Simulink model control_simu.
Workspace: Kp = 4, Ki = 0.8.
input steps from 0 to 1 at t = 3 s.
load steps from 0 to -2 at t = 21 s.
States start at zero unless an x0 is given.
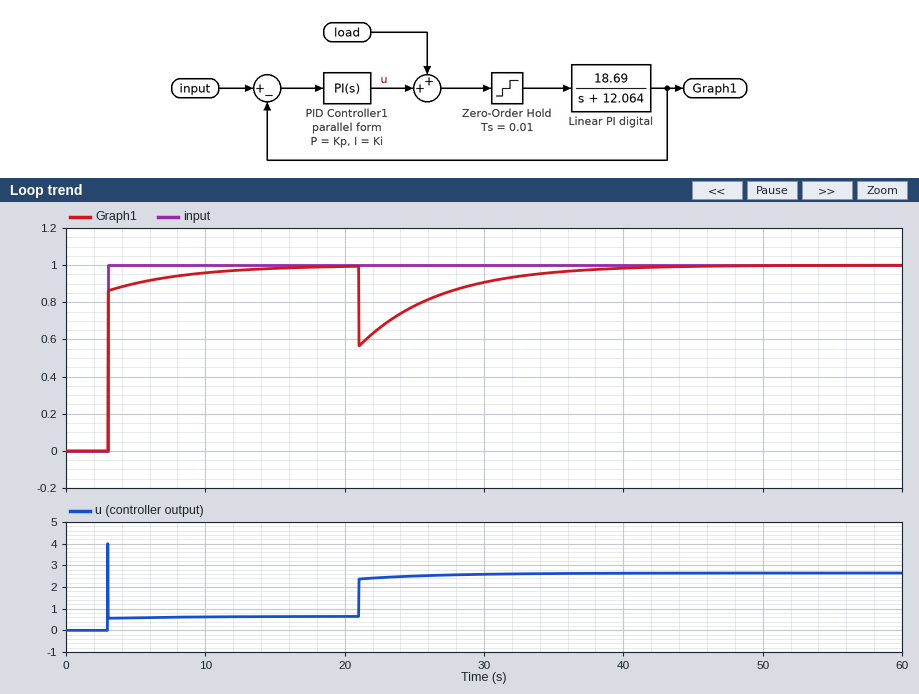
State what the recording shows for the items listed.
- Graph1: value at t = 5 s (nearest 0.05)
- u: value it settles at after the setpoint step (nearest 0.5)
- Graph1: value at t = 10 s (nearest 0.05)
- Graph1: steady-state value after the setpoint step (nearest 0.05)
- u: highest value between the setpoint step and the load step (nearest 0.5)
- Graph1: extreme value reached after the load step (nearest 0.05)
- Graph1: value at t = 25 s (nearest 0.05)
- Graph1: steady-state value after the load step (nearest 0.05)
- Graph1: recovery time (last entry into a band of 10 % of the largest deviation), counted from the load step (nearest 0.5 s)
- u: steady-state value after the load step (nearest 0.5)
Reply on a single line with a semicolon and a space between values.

0.90; 0.5; 0.95; 1.00; 4.0; 0.55; 0.80; 1.00; 13.5 s; 2.5
